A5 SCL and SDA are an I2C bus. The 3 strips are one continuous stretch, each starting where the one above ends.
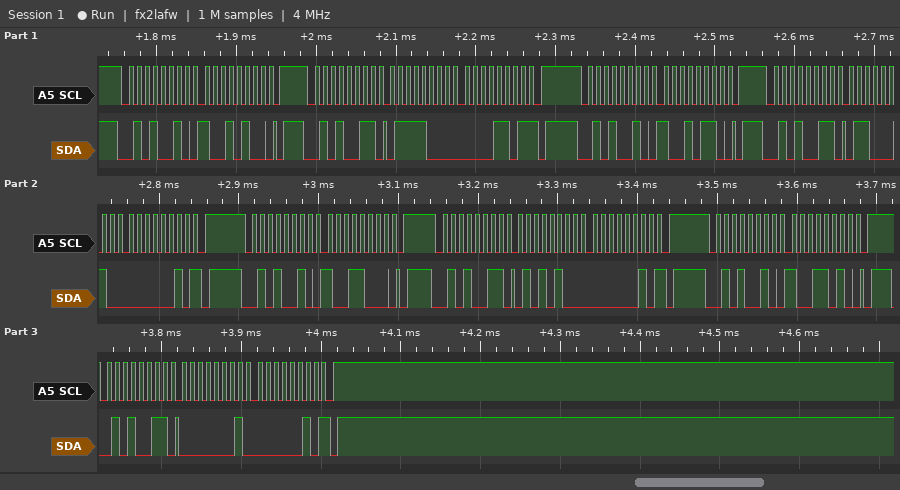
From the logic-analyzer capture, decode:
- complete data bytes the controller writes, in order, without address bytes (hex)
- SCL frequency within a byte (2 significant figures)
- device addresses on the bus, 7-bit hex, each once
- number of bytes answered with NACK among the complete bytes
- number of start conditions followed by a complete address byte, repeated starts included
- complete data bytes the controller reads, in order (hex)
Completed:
94 96 98 9A
100 kHz
0x29
4
8
78 0D 62 02 54 02 01 02
